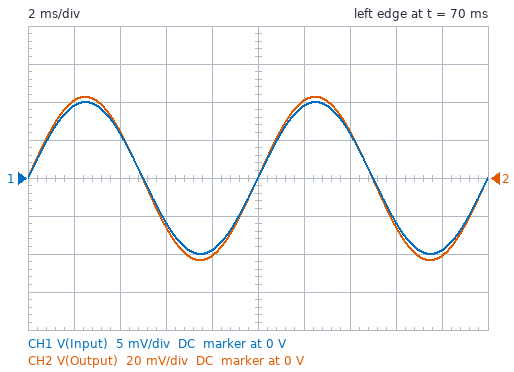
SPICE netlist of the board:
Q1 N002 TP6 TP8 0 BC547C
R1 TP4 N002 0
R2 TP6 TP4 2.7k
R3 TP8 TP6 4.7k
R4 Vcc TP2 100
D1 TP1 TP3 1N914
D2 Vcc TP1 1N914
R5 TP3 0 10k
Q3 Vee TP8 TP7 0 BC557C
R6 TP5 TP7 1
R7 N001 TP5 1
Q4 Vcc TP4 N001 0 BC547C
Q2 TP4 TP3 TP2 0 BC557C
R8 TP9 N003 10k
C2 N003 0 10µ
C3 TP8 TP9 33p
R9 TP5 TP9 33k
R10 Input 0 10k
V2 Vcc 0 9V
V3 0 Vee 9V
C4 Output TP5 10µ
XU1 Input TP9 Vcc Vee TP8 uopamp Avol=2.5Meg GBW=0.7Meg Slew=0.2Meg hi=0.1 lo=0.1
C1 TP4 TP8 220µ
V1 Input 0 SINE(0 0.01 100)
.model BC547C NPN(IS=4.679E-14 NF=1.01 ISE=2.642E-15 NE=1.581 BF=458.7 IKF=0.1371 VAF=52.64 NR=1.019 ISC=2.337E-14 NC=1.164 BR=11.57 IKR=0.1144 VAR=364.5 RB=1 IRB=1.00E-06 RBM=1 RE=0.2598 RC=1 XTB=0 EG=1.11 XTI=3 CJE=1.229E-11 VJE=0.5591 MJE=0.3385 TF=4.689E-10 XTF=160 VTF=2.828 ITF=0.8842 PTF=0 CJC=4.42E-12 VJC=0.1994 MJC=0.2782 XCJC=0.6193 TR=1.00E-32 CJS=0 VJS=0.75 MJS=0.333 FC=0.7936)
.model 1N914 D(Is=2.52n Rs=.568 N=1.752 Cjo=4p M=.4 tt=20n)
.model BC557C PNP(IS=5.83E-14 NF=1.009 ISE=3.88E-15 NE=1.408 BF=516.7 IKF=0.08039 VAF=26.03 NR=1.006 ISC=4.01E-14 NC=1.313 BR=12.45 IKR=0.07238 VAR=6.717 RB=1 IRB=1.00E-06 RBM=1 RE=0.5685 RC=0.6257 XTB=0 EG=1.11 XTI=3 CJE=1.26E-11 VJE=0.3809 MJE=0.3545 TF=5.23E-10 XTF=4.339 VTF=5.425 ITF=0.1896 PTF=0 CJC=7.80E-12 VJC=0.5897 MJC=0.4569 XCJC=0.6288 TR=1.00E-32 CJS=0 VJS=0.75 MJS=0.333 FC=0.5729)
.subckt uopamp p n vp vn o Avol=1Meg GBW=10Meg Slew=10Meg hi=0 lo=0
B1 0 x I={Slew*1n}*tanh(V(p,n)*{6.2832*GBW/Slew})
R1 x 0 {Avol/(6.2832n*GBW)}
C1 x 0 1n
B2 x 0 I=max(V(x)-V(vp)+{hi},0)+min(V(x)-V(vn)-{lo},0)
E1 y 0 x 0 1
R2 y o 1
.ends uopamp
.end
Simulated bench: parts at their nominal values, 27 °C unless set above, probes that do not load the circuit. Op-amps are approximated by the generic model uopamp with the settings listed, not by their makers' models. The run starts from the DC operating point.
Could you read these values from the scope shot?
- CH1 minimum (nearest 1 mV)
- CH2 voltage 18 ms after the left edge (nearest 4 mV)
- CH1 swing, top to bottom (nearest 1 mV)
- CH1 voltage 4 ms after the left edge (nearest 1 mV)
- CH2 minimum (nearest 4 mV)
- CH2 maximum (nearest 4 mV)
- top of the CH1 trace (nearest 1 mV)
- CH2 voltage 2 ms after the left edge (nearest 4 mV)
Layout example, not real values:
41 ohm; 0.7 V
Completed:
-10 mV; -40 mV; 20 mV; 6 mV; -44 mV; 44 mV; 10 mV; 40 mV
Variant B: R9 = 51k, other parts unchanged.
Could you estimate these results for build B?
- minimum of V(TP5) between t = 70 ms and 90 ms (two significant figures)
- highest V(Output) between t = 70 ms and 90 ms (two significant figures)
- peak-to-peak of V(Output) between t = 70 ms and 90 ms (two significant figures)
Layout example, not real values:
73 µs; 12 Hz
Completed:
-61 mV; 61 mV; 120 mV
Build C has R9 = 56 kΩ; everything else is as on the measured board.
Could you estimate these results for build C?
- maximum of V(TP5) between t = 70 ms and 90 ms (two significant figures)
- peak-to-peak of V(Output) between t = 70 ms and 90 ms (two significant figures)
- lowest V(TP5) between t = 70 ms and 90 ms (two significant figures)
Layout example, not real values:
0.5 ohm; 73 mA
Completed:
66 mV; 130 mV; -66 mV
